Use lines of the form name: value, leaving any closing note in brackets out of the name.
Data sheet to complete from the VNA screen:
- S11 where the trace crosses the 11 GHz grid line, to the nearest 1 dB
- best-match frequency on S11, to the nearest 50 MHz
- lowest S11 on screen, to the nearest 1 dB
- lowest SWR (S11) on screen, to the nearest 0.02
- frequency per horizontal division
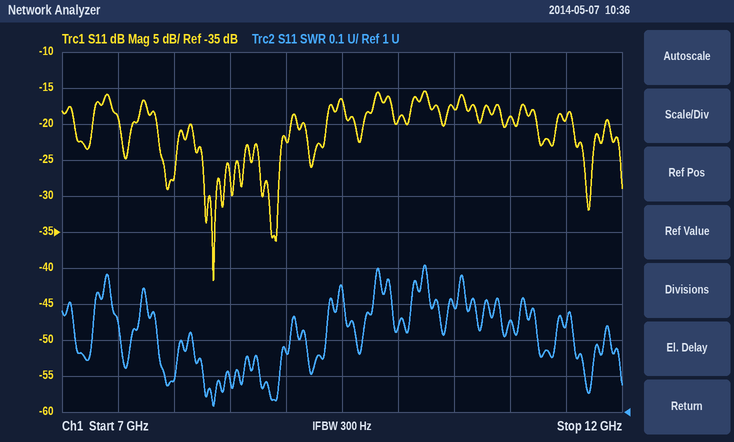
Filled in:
S11 where the trace crosses the 11 GHz grid line, to the nearest 1 dB: -19 dB
best-match frequency on S11, to the nearest 50 MHz: 8.35 GHz
lowest S11 on screen, to the nearest 1 dB: -42 dB
lowest SWR (S11) on screen, to the nearest 0.02: 1.02
frequency per horizontal division: 500 MHz
